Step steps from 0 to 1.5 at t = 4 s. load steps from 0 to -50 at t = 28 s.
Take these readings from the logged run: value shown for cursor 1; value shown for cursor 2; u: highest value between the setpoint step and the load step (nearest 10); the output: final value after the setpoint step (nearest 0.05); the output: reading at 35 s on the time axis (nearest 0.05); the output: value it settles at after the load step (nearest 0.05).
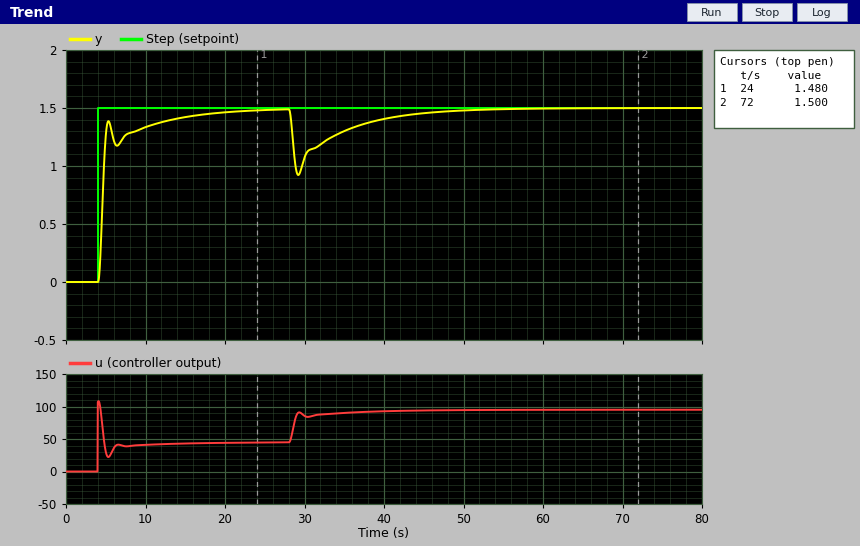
1.480
1.500
110
1.50
1.30
1.50
